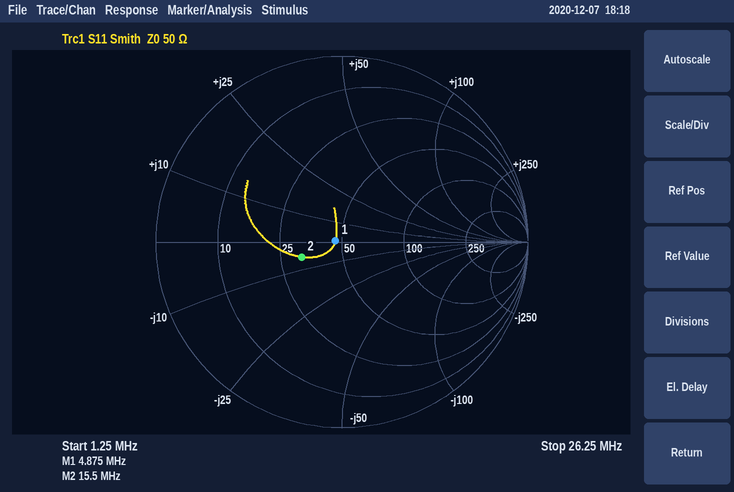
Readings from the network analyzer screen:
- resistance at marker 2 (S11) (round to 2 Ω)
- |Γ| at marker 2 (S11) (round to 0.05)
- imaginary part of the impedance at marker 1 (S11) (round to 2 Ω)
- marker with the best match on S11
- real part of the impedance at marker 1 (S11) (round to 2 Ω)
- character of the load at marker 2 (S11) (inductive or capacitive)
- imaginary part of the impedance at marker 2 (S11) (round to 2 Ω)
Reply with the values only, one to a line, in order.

32 Ω
0.25
0 Ω
marker 1
46 Ω
capacitive
-6 Ω
